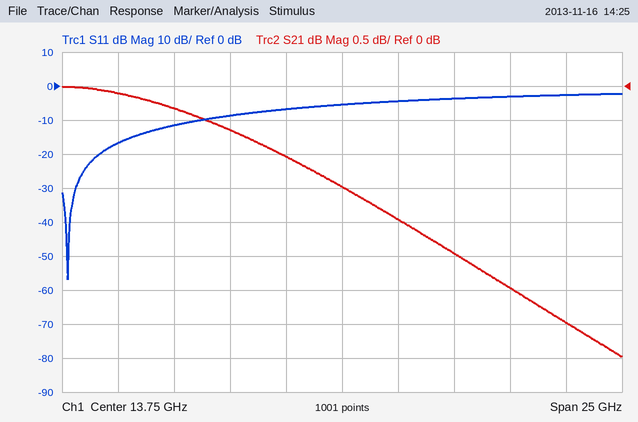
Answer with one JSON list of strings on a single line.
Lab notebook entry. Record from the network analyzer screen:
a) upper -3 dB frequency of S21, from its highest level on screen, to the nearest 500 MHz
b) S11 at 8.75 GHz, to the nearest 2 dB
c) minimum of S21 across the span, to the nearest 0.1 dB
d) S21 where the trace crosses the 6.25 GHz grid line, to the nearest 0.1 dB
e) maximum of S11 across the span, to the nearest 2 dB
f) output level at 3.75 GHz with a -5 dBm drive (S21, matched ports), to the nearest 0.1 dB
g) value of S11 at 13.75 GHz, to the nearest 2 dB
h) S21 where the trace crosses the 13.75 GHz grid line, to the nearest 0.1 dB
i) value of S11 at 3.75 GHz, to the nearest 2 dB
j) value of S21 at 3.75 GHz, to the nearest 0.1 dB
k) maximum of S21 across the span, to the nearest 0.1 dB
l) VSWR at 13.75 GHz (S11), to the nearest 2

["21.5 GHz", "-8 dB", "-4.0 dB", "-0.3 dB", "-2 dB", "-5.1 dBm", "-6 dB", "-1.5 dB", "-16 dB", "-0.1 dB", "0.0 dB", "4"]
